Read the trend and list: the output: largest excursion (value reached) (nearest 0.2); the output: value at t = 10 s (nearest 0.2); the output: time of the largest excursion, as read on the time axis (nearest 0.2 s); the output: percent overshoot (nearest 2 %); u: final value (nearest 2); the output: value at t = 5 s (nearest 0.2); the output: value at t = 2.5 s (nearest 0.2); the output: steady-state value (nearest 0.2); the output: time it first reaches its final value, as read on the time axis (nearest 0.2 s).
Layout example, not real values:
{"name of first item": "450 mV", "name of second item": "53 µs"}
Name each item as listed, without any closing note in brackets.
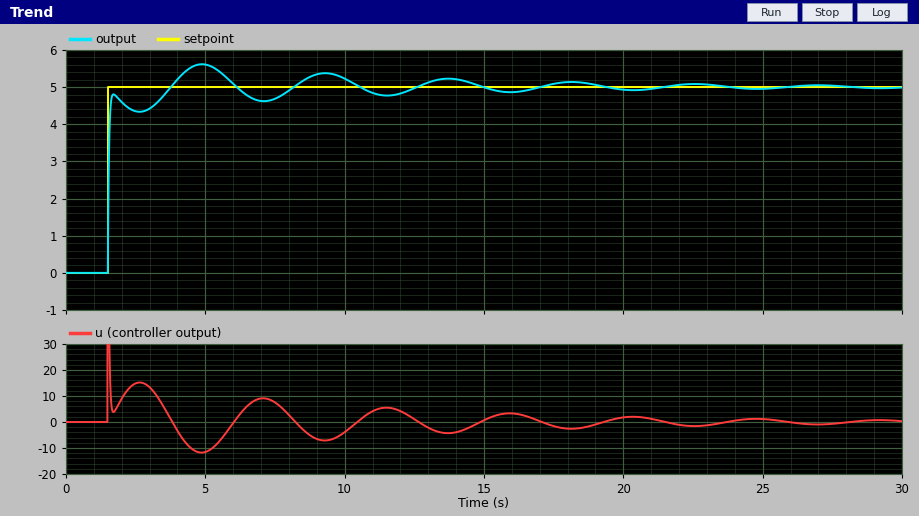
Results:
{"the output: largest excursion (value reached)": "5.6", "the output: value at t = 10 s": "5.2", "the output: time of the largest excursion, as read on the time axis": "4.8 s", "the output: percent overshoot": "12 %", "u: final value": "0", "the output: value at t = 5 s": "5.6", "the output: value at t = 2.5 s": "4.4", "the output: steady-state value": "5.0", "the output: time it first reaches its final value, as read on the time axis": "3.8 s"}
